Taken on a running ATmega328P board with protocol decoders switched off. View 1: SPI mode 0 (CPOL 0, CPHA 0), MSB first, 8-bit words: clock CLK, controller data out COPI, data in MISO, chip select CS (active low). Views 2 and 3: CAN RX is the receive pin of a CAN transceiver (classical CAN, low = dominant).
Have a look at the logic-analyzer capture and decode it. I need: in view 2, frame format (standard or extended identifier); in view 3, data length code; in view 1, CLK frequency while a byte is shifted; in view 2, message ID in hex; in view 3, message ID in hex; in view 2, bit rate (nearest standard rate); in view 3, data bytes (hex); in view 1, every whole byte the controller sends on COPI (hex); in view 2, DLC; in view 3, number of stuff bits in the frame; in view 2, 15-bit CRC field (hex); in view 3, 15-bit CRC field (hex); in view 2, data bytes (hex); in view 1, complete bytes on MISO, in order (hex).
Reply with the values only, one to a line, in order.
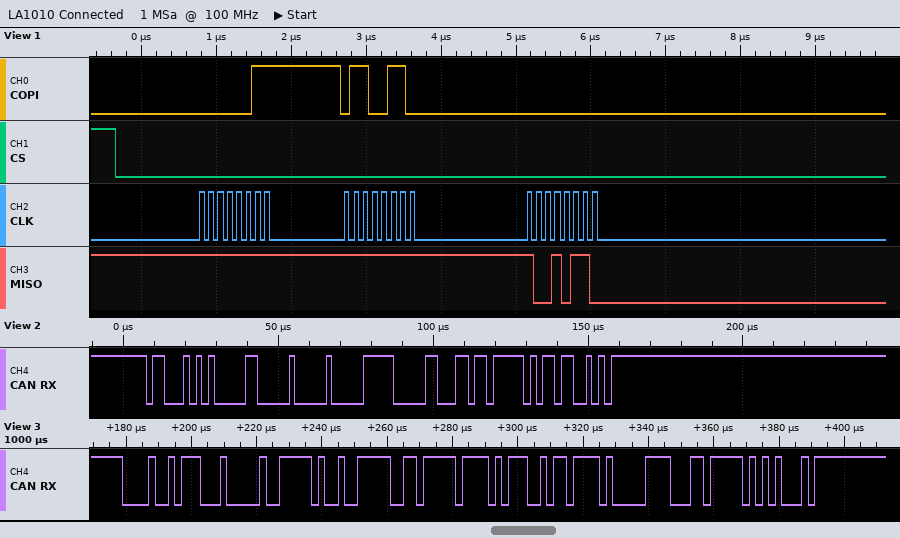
standard
8
8 MHz
0x62A
0x097
500 kbit/s
0F C9 F6 FF AE 5B D0 71
03 66 00
4
6
0x7DB2
0x5FA8
00 07 84 6D
FF FF 96
